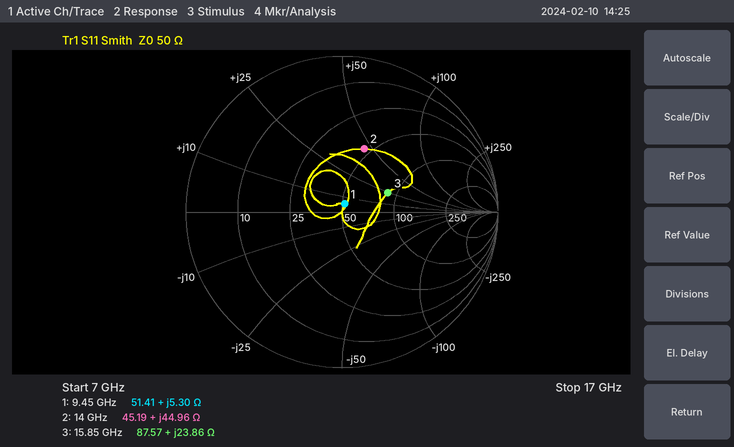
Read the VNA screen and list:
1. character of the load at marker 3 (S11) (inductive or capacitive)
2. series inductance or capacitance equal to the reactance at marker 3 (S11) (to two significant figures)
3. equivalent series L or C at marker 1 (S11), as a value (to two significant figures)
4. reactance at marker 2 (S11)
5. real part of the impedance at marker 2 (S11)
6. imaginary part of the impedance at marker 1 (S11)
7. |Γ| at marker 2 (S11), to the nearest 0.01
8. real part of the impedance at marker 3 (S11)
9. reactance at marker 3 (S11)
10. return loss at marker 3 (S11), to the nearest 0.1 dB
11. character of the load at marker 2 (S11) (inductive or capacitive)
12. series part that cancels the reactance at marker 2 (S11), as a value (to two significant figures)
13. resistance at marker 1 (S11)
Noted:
inductive
240 pH
89 pH
+44.96 Ω
45.19 Ω
+5.30 Ω
0.43
87.57 Ω
+23.86 Ω
9.9 dB
inductive
250 fF
51.41 Ω
